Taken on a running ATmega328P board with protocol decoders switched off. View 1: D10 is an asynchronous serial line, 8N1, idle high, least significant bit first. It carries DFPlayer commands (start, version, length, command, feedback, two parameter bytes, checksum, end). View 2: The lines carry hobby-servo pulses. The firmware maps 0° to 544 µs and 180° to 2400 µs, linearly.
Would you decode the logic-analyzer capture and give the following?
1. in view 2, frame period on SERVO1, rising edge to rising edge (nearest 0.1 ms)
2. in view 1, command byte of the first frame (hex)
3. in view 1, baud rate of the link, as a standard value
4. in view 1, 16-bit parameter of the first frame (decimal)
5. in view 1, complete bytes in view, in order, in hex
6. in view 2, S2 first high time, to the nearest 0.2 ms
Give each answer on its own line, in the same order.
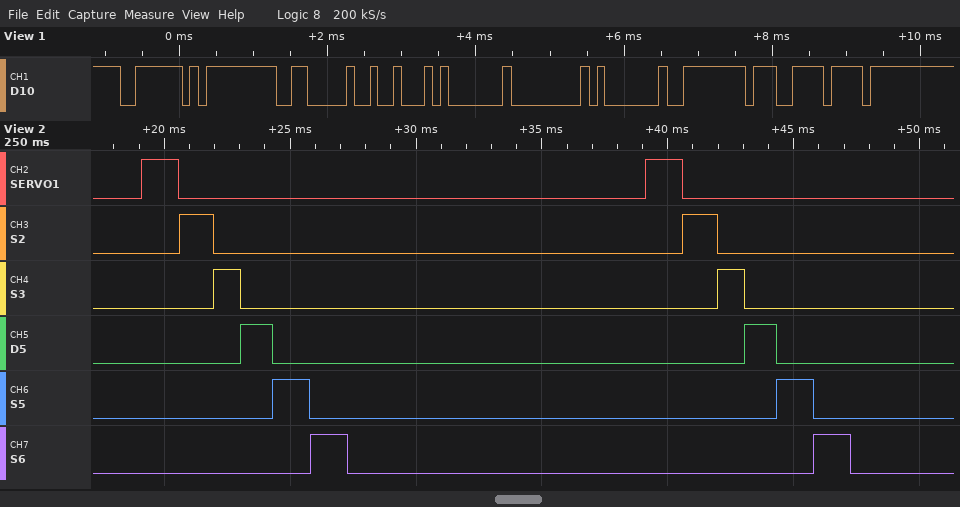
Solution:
20.0 ms
0x12
9600 baud
1
7E FF 06 12 01 00 01 FE E7 EF
1.4 ms
